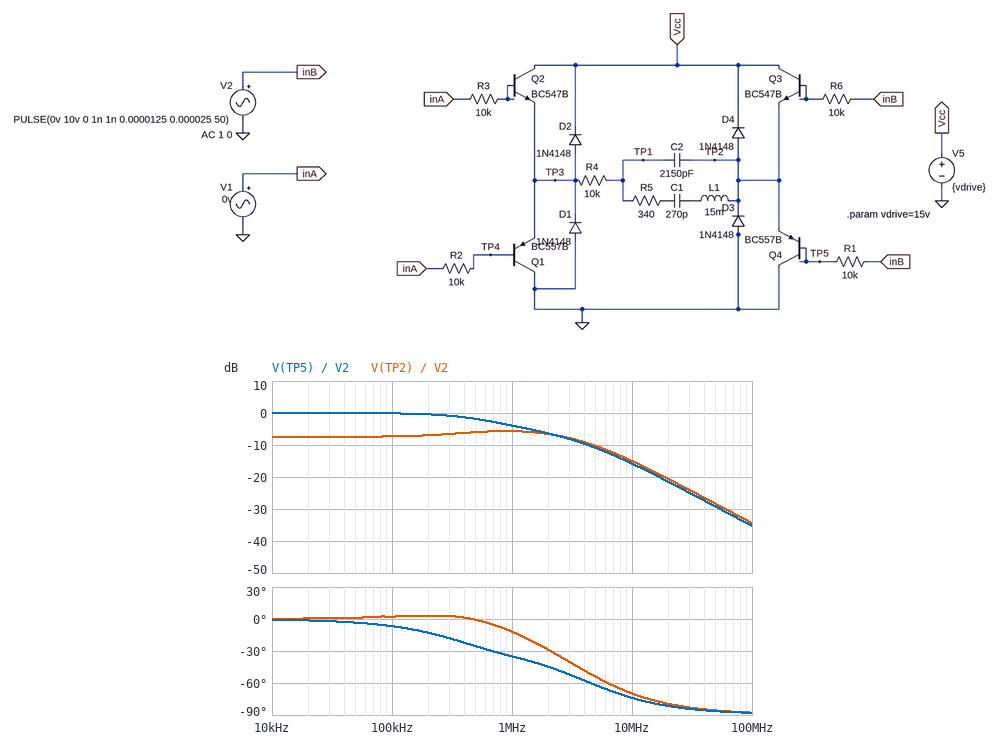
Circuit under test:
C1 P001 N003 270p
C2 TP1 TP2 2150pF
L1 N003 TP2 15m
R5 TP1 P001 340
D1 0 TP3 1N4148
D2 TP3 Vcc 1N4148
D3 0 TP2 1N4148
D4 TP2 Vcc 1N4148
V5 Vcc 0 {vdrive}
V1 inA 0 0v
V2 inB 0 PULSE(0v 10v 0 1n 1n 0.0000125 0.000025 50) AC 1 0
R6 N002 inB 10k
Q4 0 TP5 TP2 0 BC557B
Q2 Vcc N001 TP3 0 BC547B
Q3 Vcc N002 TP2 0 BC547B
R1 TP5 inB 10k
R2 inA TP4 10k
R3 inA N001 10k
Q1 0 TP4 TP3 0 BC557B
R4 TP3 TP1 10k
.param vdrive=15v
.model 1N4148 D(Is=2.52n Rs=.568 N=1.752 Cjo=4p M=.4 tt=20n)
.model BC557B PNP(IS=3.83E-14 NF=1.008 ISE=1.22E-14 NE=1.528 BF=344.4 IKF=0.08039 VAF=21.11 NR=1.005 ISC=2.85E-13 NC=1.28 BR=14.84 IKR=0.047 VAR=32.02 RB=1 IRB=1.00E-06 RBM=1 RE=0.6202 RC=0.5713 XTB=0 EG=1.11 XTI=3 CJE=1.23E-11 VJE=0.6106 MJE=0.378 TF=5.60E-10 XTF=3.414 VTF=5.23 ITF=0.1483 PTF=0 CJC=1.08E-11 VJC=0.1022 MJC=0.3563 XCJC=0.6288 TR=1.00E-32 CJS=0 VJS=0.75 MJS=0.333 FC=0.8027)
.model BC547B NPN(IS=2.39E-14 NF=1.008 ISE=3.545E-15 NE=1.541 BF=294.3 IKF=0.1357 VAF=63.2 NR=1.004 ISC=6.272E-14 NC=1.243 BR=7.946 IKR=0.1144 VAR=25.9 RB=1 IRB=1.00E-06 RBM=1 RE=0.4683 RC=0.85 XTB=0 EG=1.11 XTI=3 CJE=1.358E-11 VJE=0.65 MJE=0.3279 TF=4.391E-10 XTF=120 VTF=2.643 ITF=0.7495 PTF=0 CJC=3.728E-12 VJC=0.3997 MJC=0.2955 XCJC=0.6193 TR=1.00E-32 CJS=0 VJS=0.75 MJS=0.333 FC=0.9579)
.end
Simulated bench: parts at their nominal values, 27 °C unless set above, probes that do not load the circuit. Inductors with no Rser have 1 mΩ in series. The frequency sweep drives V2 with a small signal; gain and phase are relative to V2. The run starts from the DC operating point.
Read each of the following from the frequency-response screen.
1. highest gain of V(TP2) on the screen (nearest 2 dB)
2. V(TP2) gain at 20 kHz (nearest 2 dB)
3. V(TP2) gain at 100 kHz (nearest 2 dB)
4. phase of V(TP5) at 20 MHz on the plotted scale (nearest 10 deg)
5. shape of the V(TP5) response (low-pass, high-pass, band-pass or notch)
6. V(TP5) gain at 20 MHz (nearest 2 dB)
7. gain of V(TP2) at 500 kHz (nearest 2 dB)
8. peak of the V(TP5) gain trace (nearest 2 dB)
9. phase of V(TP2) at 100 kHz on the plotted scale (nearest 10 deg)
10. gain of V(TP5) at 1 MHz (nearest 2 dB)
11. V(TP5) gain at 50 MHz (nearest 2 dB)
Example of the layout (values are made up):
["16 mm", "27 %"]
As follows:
["-6 dB", "-8 dB", "-8 dB", "-80 deg", "low-pass", "-22 dB", "-6 dB", "0 dB", "0 deg", "-4 dB", "-30 dB"]
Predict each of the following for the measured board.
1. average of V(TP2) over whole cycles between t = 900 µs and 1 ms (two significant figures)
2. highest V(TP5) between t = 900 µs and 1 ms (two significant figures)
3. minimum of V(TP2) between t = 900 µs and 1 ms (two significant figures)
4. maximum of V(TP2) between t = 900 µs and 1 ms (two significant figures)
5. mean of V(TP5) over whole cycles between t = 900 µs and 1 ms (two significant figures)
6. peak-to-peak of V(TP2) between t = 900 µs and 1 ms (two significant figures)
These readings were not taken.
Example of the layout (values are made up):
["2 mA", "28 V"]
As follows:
["5.0 V", "10 V", "600 mV", "9.4 V", "5.0 V", "8.8 V"]
